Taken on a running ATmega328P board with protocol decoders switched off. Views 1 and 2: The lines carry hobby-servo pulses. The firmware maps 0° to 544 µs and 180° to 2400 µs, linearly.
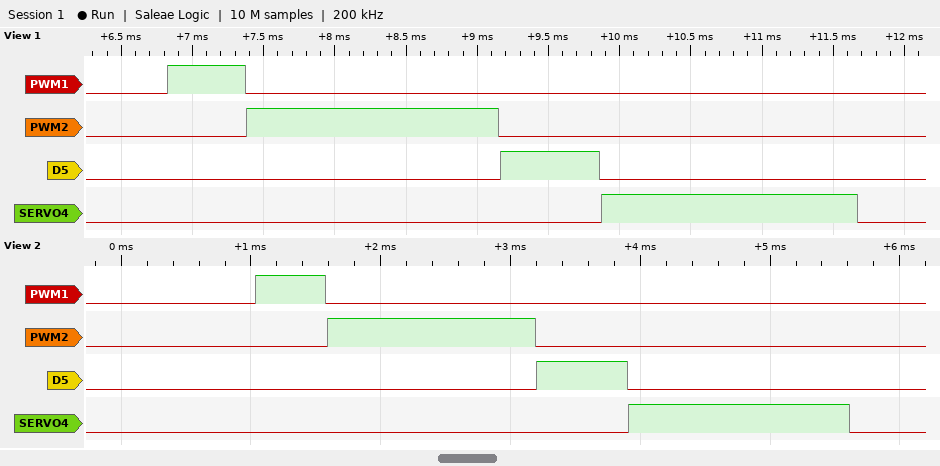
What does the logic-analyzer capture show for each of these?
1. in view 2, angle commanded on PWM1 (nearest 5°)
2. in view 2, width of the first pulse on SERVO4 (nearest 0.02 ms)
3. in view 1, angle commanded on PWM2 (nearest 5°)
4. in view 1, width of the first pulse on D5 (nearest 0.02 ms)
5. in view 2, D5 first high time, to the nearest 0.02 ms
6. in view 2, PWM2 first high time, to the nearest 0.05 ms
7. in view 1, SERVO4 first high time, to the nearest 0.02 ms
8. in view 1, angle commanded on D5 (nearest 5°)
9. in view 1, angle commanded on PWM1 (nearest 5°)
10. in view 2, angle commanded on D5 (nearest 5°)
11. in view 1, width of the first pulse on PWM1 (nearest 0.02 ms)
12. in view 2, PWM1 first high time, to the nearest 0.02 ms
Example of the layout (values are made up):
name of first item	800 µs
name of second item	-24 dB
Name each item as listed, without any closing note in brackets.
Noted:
in view 2, angle commanded on PWM1	0°
in view 2, width of the first pulse on SERVO4	1.70 ms
in view 1, angle commanded on PWM2	120°
in view 1, width of the first pulse on D5	0.70 ms
in view 2, D5 first high time, to the nearest 0.02 ms	0.70 ms
in view 2, PWM2 first high time, to the nearest 0.05 ms	1.60 ms
in view 1, SERVO4 first high time, to the nearest 0.02 ms	1.80 ms
in view 1, angle commanded on D5	15°
in view 1, angle commanded on PWM1	0°
in view 2, angle commanded on D5	15°
in view 1, width of the first pulse on PWM1	0.54 ms
in view 2, PWM1 first high time, to the nearest 0.02 ms	0.54 ms
